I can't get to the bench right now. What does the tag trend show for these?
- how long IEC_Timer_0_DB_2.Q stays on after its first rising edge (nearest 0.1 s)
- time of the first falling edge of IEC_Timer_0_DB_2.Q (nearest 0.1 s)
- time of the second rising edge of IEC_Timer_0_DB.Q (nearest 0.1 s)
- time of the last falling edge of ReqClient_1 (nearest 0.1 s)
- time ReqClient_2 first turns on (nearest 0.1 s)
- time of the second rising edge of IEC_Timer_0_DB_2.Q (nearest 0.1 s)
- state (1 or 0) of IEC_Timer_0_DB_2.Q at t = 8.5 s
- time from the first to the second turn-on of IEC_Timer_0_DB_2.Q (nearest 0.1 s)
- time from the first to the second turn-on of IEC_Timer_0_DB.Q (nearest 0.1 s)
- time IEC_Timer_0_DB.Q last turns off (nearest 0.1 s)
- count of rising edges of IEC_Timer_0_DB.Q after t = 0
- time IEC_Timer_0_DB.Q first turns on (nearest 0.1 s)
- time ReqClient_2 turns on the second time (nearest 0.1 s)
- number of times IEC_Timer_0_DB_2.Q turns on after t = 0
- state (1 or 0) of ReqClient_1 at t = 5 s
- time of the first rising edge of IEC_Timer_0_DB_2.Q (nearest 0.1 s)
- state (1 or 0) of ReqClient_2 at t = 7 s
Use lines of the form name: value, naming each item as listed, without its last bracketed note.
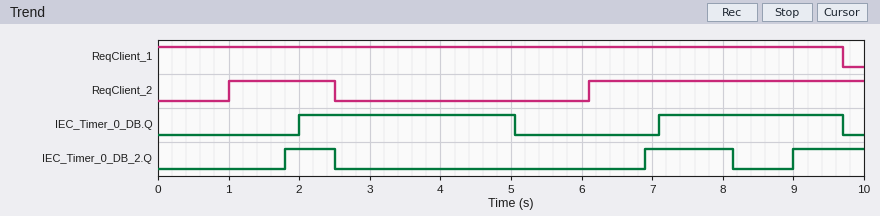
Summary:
how long IEC_Timer_0_DB_2.Q stays on after its first rising edge: 0.7 s
time of the first falling edge of IEC_Timer_0_DB_2.Q: 2.5 s
time of the second rising edge of IEC_Timer_0_DB.Q: 7.1 s
time of the last falling edge of ReqClient_1: 9.7 s
time ReqClient_2 first turns on: 1.0 s
time of the second rising edge of IEC_Timer_0_DB_2.Q: 6.9 s
state (1 or 0) of IEC_Timer_0_DB_2.Q at t = 8.5 s: 0
time from the first to the second turn-on of IEC_Timer_0_DB_2.Q: 5.1 s
time from the first to the second turn-on of IEC_Timer_0_DB.Q: 5.1 s
time IEC_Timer_0_DB.Q last turns off: 9.7 s
count of rising edges of IEC_Timer_0_DB.Q after t = 0: 2
time IEC_Timer_0_DB.Q first turns on: 2.0 s
time ReqClient_2 turns on the second time: 6.1 s
number of times IEC_Timer_0_DB_2.Q turns on after t = 0: 3
state (1 or 0) of ReqClient_1 at t = 5 s: 1
time of the first rising edge of IEC_Timer_0_DB_2.Q: 1.8 s
state (1 or 0) of ReqClient_2 at t = 7 s: 1
